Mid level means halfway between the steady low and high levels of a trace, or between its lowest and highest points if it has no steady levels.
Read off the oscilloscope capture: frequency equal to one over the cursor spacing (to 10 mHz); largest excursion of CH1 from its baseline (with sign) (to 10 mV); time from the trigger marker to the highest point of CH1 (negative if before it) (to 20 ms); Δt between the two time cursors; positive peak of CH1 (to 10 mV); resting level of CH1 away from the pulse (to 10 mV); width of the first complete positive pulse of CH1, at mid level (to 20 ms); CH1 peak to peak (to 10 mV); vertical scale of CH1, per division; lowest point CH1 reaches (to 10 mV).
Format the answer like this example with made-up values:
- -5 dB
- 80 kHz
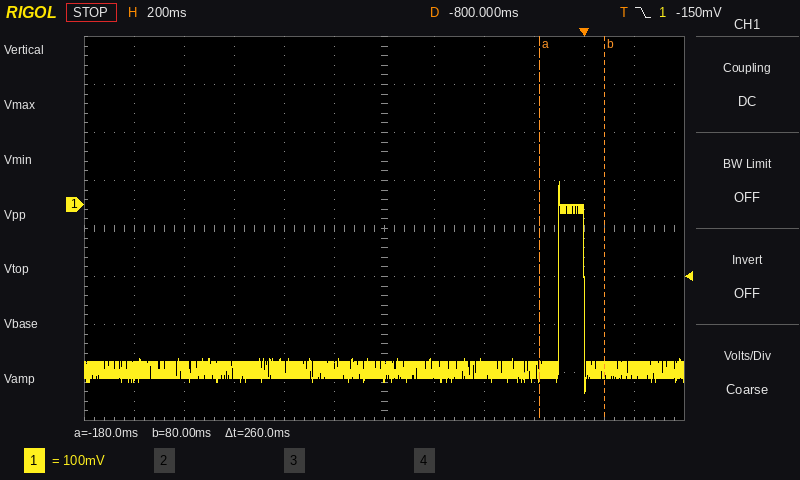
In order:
- 3.85 Hz
- +390 mV
- -100 ms
- 260 ms
- 50 mV
- -340 mV
- 100 ms
- 440 mV
- 100 mV
- -390 mV
